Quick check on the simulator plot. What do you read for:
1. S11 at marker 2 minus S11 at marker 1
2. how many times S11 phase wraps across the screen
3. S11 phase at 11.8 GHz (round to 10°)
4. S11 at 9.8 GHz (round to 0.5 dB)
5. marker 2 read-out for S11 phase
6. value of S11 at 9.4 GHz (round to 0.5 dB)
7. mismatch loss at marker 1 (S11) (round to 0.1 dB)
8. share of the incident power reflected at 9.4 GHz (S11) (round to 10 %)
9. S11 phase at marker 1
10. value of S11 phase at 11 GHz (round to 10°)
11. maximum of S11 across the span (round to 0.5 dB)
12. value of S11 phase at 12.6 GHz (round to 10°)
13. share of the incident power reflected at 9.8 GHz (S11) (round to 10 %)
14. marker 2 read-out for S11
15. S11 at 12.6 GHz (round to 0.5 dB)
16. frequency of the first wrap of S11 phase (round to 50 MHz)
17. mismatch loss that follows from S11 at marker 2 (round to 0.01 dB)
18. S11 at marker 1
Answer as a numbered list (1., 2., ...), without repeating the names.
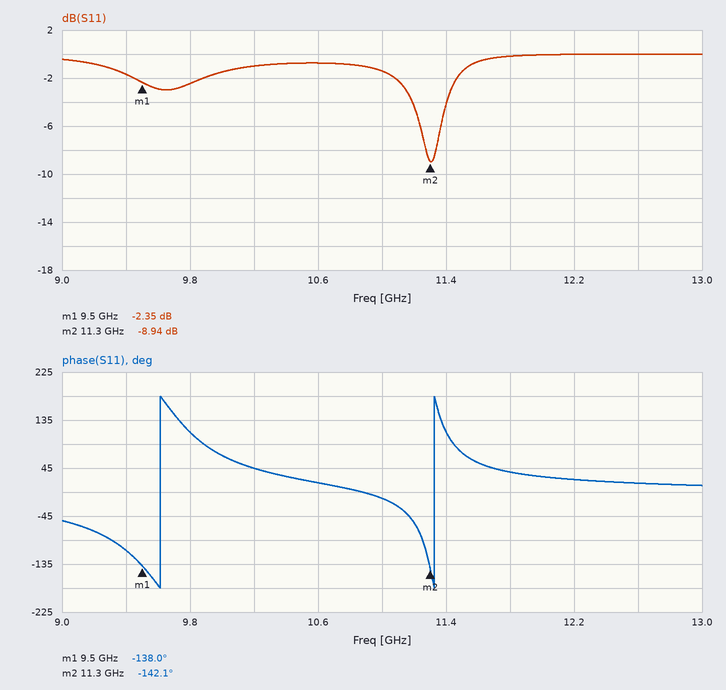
1. -6.59 dB
2. 2
3. 40°
4. -2.5 dB
5. -142.1°
6. -1.5 dB
7. 3.8 dB
8. 70 %
9. -138.0°
10. -10°
11. 0.0 dB
12. 20°
13. 60 %
14. -8.94 dB
15. 0.0 dB
16. 9.60 GHz
17. 0.59 dB
18. -2.35 dB
